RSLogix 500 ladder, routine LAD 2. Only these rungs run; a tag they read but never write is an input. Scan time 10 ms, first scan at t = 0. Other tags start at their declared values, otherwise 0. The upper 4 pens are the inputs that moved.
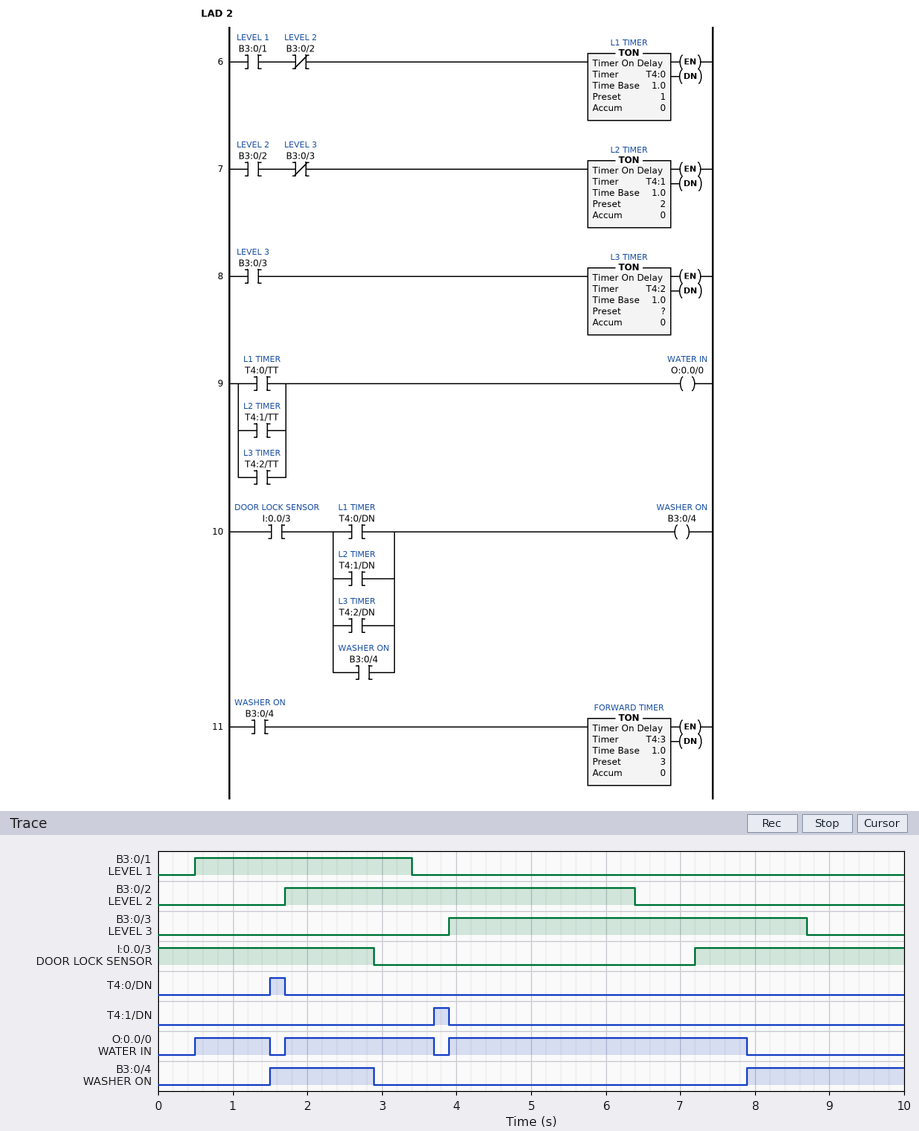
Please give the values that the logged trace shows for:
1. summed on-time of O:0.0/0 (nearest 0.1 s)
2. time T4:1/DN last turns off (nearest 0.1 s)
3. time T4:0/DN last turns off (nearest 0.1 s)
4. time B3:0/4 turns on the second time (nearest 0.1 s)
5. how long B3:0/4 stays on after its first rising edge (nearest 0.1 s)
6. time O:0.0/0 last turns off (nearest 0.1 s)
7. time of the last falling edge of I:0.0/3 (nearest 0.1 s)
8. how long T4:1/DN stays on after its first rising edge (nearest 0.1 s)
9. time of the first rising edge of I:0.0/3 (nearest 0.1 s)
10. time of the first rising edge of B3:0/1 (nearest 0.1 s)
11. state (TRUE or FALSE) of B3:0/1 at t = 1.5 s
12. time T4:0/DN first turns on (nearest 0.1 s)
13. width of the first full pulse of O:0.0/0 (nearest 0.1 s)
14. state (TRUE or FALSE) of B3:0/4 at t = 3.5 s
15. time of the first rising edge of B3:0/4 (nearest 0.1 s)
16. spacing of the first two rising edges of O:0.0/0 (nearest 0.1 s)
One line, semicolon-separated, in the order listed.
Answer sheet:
7.0 s; 3.9 s; 1.7 s; 7.9 s; 1.4 s; 7.9 s; 2.9 s; 0.2 s; 7.2 s; 0.5 s; TRUE; 1.5 s; 1.0 s; FALSE; 1.5 s; 1.2 s
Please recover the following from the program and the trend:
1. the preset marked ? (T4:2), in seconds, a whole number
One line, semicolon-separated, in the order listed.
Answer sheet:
4 s
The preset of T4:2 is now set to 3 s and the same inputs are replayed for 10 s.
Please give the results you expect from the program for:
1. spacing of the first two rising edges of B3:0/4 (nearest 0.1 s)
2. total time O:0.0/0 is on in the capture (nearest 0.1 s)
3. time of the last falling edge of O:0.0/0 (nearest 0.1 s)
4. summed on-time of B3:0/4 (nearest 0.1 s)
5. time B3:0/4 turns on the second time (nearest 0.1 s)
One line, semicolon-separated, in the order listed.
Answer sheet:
5.7 s; 6.0 s; 6.9 s; 4.2 s; 7.2 s
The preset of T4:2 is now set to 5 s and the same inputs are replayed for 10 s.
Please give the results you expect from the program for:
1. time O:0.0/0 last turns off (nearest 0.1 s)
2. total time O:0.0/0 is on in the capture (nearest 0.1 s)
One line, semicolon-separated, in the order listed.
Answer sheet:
8.7 s; 7.8 s
